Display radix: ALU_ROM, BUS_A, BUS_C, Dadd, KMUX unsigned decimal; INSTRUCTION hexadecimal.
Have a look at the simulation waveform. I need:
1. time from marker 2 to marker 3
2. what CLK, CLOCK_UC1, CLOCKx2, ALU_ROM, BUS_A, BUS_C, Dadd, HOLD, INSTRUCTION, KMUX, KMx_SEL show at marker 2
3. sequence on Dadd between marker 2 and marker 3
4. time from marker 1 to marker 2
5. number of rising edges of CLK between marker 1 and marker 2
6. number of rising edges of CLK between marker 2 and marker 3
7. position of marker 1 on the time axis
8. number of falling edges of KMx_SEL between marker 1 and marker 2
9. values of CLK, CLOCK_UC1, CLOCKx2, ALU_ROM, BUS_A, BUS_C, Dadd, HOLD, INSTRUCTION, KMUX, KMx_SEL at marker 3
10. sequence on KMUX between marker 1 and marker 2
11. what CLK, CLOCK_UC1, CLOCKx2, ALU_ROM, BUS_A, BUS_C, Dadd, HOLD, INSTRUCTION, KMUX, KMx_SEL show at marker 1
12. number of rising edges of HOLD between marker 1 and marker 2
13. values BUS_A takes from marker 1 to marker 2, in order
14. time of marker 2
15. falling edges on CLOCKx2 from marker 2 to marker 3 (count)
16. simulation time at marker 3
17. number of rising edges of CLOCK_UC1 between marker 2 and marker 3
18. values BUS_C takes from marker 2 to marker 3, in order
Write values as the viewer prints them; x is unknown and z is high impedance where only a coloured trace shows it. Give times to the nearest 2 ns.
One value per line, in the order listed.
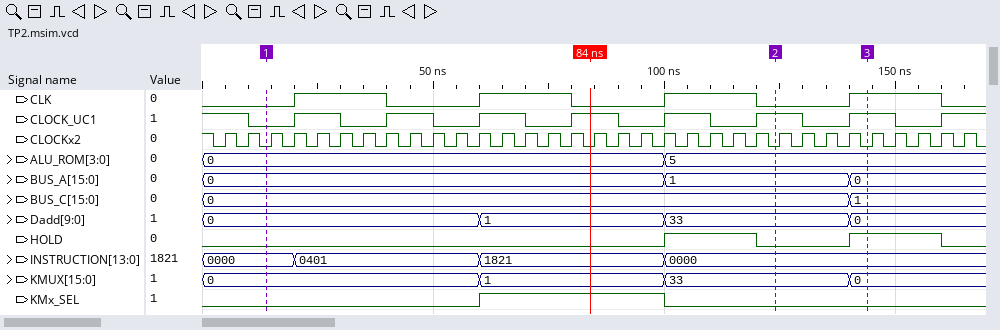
20 ns
CLK=0, CLOCK_UC1=1, CLOCKx2=0, ALU_ROM=5, BUS_A=1, BUS_C=0, Dadd=33, HOLD=0, INSTRUCTION=0000, KMUX=33, KMx_SEL=0
33, 0
110 ns
3
1
14 ns
1
CLK=1, CLOCK_UC1=1, CLOCKx2=0, ALU_ROM=5, BUS_A=0, BUS_C=1, Dadd=0, HOLD=1, INSTRUCTION=0000, KMUX=0, KMx_SEL=0
0, 1, 33
CLK=0, CLOCK_UC1=0, CLOCKx2=0, ALU_ROM=0, BUS_A=0, BUS_C=0, Dadd=0, HOLD=0, INSTRUCTION=0000, KMUX=0, KMx_SEL=0
1
0, 1
124 ns
4
144 ns
1
0, 1
